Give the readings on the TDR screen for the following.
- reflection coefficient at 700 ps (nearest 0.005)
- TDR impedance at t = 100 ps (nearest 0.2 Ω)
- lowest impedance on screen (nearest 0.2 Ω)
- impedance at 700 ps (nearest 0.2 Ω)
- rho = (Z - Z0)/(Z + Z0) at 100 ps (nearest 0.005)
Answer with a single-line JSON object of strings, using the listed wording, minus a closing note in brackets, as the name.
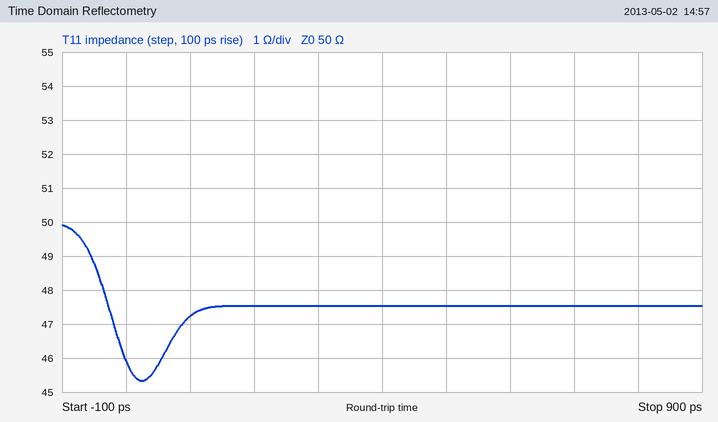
{"reflection coefficient at 700 ps": "-0.025", "TDR impedance at t = 100 ps": "47.2 Ω", "lowest impedance on screen": "45.4 Ω", "impedance at 700 ps": "47.6 Ω", "rho = (Z - Z0)/(Z + Z0) at 100 ps": "-0.030"}
